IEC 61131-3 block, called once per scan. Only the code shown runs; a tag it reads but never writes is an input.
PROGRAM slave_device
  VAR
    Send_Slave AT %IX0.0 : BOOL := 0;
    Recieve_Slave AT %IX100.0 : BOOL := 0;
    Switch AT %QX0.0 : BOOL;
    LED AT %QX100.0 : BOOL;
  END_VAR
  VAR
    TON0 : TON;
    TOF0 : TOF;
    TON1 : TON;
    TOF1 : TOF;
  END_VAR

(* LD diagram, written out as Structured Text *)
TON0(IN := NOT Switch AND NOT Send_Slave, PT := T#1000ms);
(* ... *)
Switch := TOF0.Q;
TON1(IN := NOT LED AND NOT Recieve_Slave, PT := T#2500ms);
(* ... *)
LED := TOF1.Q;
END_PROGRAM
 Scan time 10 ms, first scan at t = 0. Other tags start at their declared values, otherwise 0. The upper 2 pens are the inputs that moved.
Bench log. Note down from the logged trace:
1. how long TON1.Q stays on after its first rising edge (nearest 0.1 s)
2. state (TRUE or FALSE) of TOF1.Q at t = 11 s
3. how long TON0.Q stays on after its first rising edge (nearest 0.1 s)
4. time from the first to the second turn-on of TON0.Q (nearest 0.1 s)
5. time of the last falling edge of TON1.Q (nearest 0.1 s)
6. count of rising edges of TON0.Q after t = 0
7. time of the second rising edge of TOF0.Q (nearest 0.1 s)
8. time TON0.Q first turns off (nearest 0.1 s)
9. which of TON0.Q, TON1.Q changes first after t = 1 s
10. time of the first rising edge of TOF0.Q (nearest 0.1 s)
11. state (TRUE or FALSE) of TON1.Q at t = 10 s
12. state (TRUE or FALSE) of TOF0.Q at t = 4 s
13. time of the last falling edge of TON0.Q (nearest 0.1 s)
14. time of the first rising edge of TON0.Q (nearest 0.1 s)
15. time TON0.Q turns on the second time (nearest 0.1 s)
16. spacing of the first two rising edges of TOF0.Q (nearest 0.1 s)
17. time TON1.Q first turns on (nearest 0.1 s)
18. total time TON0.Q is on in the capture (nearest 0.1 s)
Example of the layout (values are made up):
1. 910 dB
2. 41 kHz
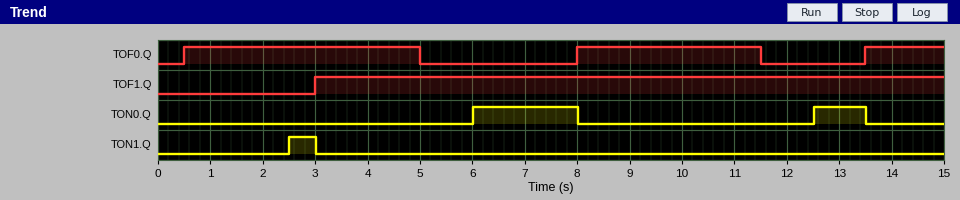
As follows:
1. 0.5 s
2. TRUE
3. 2.0 s
4. 6.5 s
5. 3.0 s
6. 2
7. 8.0 s
8. 8.0 s
9. TON1.Q
10. 0.5 s
11. FALSE
12. TRUE
13. 13.5 s
14. 6.0 s
15. 12.5 s
16. 7.5 s
17. 2.5 s
18. 3.0 s
